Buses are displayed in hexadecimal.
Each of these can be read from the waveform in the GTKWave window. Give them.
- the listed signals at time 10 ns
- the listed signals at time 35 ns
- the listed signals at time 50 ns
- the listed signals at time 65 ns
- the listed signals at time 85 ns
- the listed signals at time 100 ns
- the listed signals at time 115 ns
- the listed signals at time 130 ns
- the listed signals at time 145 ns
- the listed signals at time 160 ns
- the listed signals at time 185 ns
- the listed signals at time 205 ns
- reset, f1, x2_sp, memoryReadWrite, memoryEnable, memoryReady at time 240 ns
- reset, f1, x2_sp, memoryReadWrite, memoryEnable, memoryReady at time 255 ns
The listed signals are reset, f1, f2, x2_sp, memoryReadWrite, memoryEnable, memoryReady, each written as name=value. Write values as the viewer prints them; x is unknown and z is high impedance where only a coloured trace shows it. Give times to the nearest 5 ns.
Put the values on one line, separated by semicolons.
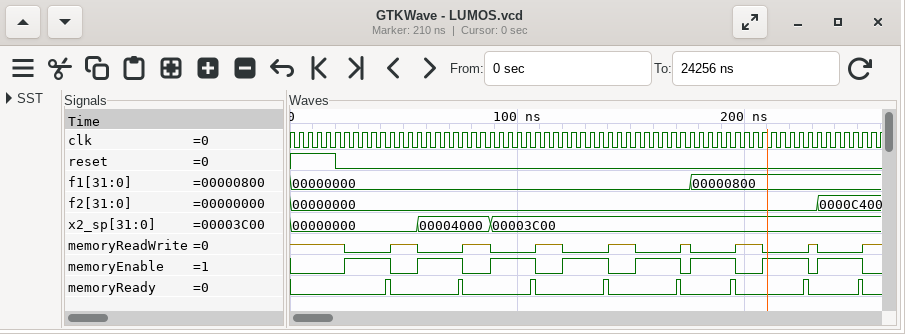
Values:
reset=1, f1=00000000, f2=00000000, x2_sp=00000000, memoryReadWrite=z, memoryEnable=0, memoryReady=0; reset=0, f1=00000000, f2=00000000, x2_sp=00000000, memoryReadWrite=0, memoryEnable=1, memoryReady=0; reset=0, f1=00000000, f2=00000000, x2_sp=00000000, memoryReadWrite=z, memoryEnable=0, memoryReady=0; reset=0, f1=00000000, f2=00000000, x2_sp=00004000, memoryReadWrite=0, memoryEnable=1, memoryReady=0; reset=0, f1=00000000, f2=00000000, x2_sp=00004000, memoryReadWrite=z, memoryEnable=0, memoryReady=0; reset=0, f1=00000000, f2=00000000, x2_sp=00003C00, memoryReadWrite=0, memoryEnable=1, memoryReady=0; reset=0, f1=00000000, f2=00000000, x2_sp=00003C00, memoryReadWrite=z, memoryEnable=0, memoryReady=0; reset=0, f1=00000000, f2=00000000, x2_sp=00003C00, memoryReadWrite=0, memoryEnable=1, memoryReady=0; reset=0, f1=00000000, f2=00000000, x2_sp=00003C00, memoryReadWrite=z, memoryEnable=0, memoryReady=0; reset=0, f1=00000000, f2=00000000, x2_sp=00003C00, memoryReadWrite=0, memoryEnable=1, memoryReady=0; reset=0, f1=00000800, f2=00000000, x2_sp=00003C00, memoryReadWrite=0, memoryEnable=1, memoryReady=0; reset=0, f1=00000800, f2=00000000, x2_sp=00003C00, memoryReadWrite=z, memoryEnable=0, memoryReady=0; reset=0, f1=00000800, x2_sp=00003C00, memoryReadWrite=0, memoryEnable=1, memoryReady=0; reset=0, f1=00000800, x2_sp=00003C00, memoryReadWrite=z, memoryEnable=0, memoryReady=0
